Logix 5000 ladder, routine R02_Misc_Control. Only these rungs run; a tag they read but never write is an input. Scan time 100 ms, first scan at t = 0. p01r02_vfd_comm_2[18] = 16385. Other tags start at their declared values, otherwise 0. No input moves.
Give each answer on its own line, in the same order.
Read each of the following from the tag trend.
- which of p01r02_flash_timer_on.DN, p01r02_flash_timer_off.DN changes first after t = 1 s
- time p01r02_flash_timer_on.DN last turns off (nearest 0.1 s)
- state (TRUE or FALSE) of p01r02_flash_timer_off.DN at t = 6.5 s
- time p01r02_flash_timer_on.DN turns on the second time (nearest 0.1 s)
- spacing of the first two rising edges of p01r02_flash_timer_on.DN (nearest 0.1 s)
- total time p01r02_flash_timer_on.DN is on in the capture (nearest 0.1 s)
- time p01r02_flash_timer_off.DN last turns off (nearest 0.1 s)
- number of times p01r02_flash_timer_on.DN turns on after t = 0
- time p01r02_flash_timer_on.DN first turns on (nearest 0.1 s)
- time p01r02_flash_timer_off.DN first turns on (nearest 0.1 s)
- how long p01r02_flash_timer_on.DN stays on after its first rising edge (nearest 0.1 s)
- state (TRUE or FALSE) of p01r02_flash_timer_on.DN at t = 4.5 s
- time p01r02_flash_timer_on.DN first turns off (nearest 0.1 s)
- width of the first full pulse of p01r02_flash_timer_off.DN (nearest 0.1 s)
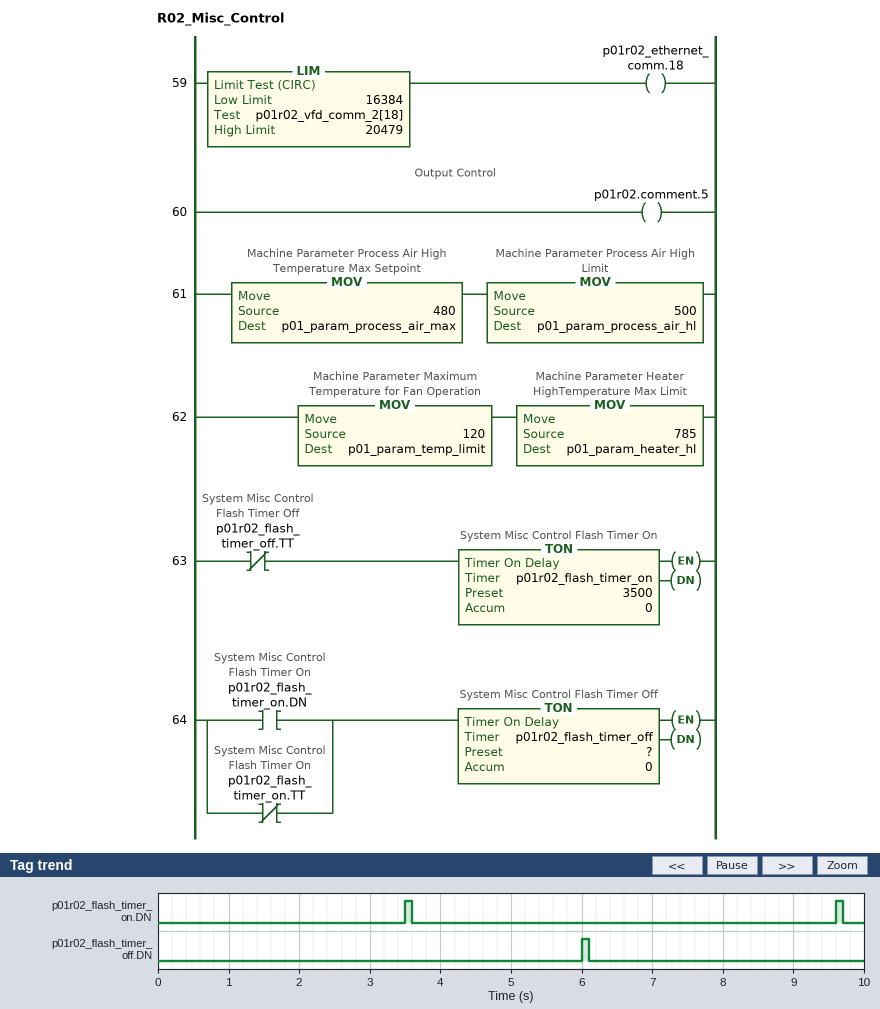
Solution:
p01r02_flash_timer_on.DN
9.7 s
FALSE
9.6 s
6.1 s
0.2 s
6.1 s
2
3.5 s
6.0 s
0.1 s
FALSE
3.6 s
0.1 s
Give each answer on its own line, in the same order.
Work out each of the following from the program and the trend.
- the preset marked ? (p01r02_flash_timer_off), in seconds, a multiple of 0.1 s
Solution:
2.5 s
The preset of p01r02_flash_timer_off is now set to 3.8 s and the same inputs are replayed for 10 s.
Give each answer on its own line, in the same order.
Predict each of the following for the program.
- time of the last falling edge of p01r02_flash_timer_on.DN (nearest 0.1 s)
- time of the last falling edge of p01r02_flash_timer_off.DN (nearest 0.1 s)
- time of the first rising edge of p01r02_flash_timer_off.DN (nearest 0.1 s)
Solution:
3.6 s
7.4 s
7.3 s
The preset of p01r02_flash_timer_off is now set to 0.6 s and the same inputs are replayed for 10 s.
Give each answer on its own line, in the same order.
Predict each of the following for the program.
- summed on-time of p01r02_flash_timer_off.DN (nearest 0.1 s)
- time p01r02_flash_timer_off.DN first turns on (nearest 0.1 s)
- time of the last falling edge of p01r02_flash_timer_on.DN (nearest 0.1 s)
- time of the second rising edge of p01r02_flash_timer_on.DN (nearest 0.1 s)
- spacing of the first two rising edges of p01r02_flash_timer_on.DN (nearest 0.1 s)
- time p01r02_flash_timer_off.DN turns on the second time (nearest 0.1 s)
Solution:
0.2 s
4.1 s
7.8 s
7.7 s
4.2 s
8.3 s
